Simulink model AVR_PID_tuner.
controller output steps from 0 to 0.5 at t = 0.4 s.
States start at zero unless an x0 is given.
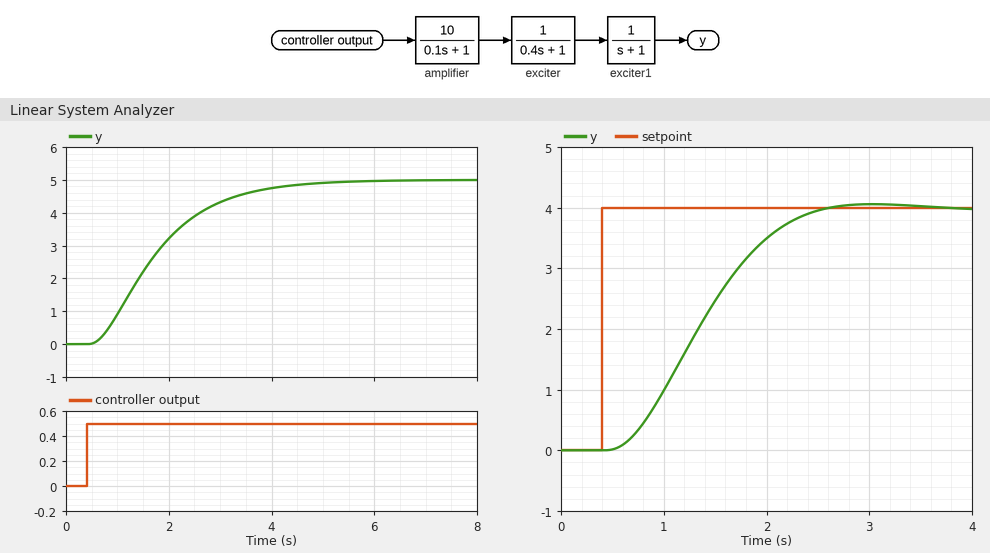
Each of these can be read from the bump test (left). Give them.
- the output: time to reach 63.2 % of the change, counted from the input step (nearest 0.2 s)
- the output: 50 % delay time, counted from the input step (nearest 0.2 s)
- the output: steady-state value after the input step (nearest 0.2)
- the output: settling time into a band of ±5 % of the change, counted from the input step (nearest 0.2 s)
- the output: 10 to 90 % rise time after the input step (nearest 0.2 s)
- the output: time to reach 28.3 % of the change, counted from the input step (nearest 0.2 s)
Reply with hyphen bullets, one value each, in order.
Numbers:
- 1.6 s
- 1.2 s
- 5.0
- 3.6 s
- 2.4 s
- 0.8 s
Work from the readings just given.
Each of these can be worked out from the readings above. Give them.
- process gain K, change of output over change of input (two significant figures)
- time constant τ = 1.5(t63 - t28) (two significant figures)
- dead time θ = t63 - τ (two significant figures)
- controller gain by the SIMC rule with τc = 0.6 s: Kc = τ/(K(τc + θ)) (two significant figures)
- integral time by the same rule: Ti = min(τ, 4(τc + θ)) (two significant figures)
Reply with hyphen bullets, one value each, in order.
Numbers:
- 10
- 1.2 s
- 0.40 s
- 0.12
- 1.2 s
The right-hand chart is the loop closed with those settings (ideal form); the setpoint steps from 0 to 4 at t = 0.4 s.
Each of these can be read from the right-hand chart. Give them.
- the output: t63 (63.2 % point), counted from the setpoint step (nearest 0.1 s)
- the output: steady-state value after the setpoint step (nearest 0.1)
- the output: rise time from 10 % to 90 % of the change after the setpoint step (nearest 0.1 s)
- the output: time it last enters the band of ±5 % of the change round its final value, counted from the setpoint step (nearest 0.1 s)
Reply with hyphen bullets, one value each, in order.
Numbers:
- 1.1 s
- 4.0
- 1.3 s
- 1.9 s
